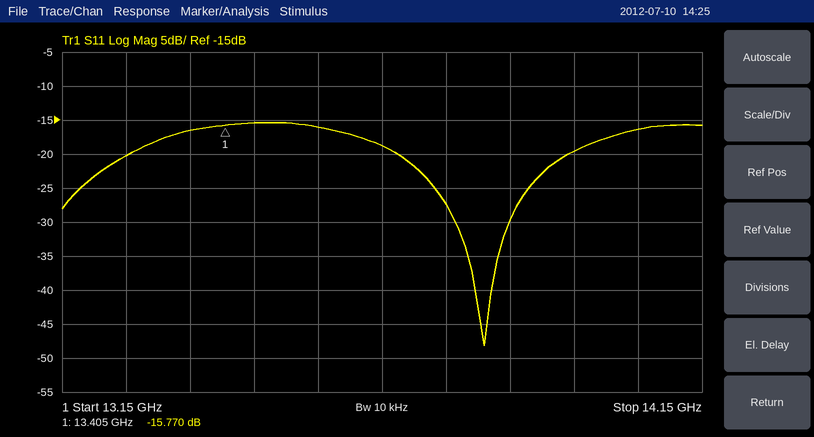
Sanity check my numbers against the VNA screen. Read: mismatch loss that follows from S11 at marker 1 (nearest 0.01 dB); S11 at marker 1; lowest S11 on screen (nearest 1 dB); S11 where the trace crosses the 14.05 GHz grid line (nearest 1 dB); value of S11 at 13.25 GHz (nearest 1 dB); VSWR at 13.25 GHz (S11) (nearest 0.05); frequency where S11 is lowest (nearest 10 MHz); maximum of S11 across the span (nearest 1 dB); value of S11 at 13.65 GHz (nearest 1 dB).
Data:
0.12 dB
-15.770 dB
-48 dB
-16 dB
-20 dB
1.20
13.81 GHz
-15 dB
-19 dB
